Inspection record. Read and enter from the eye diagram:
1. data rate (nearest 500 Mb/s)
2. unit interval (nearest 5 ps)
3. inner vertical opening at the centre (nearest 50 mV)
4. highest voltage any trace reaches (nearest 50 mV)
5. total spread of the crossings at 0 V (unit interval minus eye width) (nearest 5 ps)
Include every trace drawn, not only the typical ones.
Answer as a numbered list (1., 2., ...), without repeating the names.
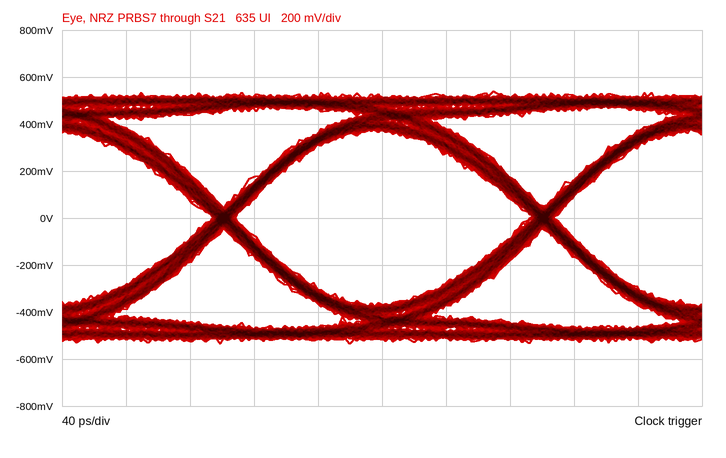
1. 5.0 Gb/s
2. 200 ps
3. 750 mV
4. 550 mV
5. 15 ps
